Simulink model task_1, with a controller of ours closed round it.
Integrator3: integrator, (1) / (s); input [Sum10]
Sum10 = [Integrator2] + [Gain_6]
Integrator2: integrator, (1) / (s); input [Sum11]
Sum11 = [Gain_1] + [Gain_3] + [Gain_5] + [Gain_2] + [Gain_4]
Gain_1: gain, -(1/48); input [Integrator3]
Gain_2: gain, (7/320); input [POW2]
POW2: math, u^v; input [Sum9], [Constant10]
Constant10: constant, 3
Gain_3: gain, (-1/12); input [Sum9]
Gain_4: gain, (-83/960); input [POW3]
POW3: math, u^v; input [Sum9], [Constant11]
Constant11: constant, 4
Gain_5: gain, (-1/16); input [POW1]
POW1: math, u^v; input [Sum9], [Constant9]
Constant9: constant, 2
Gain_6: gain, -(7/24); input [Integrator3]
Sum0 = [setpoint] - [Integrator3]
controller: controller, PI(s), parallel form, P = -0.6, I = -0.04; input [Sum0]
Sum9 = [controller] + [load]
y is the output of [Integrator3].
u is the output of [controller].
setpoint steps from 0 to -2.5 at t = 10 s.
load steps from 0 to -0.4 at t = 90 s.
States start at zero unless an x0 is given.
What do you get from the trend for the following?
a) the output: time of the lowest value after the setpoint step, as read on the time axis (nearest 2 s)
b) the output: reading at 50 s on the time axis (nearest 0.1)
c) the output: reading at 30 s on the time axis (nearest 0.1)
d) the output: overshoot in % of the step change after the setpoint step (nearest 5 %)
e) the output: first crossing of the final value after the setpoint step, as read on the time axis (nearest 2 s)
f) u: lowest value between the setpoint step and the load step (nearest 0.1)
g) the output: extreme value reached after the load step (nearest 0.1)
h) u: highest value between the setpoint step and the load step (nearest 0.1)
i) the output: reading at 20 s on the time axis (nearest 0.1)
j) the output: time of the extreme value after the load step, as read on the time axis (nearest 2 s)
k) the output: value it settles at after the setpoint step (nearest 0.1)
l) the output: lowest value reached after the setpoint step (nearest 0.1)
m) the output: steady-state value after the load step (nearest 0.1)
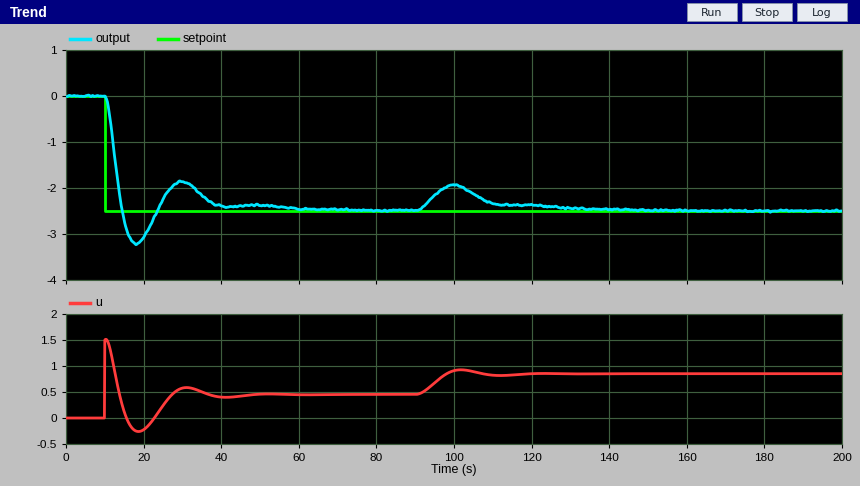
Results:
18 s
-2.4
-1.9
30 %
14 s
-0.3
-1.9
1.5
-3.1
100 s
-2.5
-3.2
-2.5
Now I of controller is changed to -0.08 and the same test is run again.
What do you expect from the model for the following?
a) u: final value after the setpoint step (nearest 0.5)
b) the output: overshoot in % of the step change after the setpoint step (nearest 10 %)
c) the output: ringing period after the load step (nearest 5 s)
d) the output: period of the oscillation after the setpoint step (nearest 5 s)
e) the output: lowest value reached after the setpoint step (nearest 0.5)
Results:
0.5
50 %
20 s
25 s
-3.5
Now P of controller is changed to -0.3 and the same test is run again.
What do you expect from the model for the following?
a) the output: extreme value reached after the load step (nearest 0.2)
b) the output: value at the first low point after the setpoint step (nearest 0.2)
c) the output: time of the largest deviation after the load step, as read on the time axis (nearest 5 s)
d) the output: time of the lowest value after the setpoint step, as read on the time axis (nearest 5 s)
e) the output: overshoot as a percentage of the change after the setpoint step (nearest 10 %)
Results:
-1.8
-3.0
100 s
25 s
20 %
